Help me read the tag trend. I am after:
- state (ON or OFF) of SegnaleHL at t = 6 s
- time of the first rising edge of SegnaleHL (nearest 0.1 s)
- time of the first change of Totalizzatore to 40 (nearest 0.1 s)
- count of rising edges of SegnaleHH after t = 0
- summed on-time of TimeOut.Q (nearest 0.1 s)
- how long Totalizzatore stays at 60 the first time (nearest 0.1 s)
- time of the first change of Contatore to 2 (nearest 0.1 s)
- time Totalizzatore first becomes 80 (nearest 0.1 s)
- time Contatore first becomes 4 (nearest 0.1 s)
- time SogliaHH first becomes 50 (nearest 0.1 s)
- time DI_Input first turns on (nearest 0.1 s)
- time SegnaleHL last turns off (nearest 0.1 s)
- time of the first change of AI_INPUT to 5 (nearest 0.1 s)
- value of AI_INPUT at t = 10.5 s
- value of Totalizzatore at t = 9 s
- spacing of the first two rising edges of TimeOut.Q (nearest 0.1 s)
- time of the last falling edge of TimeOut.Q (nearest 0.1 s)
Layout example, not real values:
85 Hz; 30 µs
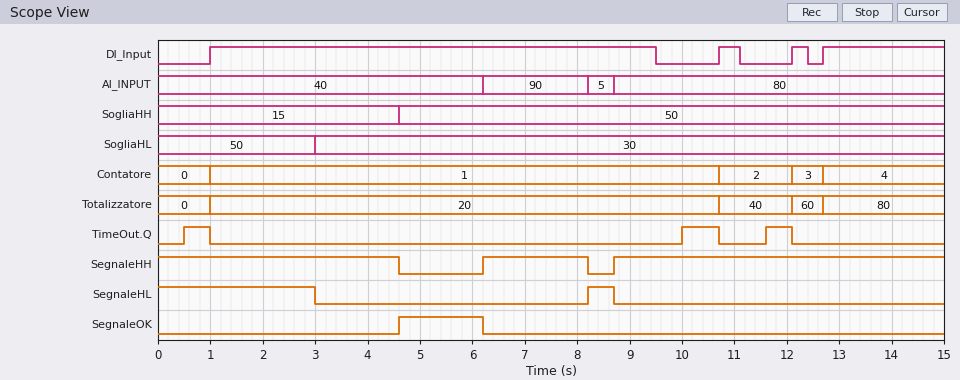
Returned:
OFF; 8.2 s; 10.7 s; 2; 1.7 s; 0.6 s; 10.7 s; 12.7 s; 12.7 s; 4.6 s; 1.0 s; 8.7 s; 8.2 s; 80; 20; 9.5 s; 12.1 s
